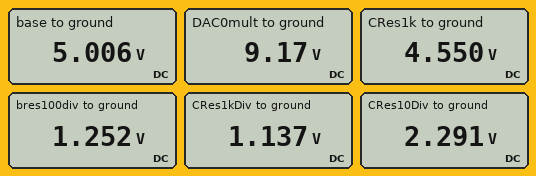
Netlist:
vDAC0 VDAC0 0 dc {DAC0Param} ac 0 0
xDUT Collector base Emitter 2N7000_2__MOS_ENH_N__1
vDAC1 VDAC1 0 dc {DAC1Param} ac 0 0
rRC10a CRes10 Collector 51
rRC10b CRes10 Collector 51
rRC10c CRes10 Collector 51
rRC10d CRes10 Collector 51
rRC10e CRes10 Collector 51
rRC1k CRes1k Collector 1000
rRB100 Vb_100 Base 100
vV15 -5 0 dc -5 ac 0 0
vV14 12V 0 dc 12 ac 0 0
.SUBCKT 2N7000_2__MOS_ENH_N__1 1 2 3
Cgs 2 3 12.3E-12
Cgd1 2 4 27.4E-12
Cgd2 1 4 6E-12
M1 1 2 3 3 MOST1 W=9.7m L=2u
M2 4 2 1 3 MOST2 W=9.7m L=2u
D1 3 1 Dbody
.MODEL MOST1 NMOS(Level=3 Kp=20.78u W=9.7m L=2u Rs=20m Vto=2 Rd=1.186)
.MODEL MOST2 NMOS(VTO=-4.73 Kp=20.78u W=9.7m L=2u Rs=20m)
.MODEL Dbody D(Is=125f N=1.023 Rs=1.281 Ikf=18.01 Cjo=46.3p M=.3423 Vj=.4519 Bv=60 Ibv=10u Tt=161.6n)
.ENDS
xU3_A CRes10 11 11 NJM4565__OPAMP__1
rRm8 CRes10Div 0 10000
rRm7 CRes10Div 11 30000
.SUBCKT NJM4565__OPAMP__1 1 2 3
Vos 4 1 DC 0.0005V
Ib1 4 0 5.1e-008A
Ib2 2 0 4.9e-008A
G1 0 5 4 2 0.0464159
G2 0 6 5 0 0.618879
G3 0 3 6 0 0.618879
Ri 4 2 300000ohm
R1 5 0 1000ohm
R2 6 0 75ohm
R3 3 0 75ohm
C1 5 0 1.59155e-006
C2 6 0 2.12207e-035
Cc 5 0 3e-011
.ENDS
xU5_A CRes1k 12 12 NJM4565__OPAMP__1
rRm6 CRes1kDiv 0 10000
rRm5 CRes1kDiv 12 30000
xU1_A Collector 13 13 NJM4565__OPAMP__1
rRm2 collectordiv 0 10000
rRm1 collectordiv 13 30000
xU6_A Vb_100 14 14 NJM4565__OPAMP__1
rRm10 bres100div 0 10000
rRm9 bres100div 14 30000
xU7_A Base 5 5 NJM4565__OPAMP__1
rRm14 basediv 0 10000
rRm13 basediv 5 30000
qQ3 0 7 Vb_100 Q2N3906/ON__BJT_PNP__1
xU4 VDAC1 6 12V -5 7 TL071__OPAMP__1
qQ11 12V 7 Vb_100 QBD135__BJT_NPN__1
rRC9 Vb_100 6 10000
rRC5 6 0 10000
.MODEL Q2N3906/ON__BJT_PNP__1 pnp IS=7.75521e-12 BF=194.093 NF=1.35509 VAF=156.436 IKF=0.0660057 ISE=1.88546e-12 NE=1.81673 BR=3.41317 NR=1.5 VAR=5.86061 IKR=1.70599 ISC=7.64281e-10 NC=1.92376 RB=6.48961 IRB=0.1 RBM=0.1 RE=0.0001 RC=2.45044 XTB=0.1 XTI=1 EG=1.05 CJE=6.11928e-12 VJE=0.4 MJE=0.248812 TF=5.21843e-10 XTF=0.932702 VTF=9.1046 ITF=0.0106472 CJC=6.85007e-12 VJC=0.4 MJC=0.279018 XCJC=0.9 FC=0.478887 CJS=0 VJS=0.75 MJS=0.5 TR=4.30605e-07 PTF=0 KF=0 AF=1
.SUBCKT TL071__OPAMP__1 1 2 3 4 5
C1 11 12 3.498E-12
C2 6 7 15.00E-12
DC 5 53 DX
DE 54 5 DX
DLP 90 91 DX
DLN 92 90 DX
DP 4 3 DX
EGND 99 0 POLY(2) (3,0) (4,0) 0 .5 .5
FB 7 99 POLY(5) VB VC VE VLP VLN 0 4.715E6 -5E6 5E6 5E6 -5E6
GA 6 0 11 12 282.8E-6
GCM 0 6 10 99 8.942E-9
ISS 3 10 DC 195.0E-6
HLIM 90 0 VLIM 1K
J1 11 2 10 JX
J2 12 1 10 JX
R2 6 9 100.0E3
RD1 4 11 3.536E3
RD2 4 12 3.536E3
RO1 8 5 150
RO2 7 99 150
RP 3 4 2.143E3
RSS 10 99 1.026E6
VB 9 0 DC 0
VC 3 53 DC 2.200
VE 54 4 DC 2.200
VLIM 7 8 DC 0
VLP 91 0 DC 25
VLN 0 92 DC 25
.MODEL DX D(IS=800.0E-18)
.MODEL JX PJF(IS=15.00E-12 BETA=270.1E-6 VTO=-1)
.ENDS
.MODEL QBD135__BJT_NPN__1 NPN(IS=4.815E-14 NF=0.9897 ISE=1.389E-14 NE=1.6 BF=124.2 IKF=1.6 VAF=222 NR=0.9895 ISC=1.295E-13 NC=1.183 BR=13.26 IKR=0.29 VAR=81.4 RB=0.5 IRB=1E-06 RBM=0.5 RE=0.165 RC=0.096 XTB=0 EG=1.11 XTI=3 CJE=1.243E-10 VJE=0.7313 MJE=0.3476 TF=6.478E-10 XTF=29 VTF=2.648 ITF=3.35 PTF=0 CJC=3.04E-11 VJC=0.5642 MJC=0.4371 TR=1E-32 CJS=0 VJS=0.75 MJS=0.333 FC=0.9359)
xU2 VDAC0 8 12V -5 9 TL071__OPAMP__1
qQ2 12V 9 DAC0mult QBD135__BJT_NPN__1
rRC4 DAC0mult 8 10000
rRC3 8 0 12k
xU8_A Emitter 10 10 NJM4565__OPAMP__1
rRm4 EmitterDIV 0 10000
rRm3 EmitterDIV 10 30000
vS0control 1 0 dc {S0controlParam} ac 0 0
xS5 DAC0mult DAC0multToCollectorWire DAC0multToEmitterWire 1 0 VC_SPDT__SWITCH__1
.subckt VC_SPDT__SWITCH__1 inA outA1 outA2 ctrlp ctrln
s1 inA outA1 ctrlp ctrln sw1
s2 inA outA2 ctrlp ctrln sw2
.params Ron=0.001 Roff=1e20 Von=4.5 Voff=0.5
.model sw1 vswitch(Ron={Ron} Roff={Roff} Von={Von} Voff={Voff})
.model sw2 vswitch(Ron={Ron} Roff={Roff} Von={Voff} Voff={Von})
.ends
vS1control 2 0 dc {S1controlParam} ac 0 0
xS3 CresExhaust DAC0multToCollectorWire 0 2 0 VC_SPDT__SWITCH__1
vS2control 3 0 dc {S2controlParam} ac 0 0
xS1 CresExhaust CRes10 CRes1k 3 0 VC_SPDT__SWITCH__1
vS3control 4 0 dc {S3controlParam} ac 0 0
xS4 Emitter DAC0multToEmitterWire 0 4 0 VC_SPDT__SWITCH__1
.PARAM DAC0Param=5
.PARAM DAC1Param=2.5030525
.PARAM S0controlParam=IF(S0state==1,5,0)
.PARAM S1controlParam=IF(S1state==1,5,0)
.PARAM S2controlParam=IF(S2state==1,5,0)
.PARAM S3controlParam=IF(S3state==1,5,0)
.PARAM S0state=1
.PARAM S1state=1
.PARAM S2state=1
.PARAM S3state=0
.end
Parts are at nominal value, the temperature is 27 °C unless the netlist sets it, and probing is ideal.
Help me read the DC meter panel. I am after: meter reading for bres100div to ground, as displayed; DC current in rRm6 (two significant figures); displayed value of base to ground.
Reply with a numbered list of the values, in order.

1. 1.252 V
2. 110 µA
3. 5.006 V
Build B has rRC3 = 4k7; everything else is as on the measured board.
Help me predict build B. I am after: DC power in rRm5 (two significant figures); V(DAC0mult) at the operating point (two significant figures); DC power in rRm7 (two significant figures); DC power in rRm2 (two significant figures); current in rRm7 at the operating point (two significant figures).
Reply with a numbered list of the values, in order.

1. 470 µW
2. 9.6 V
3. 1.7 mW
4. 160 µW
5. 240 µA
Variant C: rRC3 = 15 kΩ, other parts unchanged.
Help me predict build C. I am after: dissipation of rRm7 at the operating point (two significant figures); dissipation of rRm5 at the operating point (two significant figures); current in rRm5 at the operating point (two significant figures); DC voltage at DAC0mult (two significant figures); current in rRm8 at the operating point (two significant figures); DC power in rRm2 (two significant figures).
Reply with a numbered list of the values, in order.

1. 1.3 mW
2. 260 µW
3. 93 µA
4. 8.3 V
5. 210 µA
6. 86 µW
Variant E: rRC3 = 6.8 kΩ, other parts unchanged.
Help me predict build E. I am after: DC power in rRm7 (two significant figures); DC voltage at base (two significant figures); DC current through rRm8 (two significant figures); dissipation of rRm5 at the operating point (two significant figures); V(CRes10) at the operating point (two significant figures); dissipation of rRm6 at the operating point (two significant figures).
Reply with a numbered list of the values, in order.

1. 1.7 mW
2. 5.0 V
3. 240 µA
4. 470 µW
5. 9.6 V
6. 160 µW
